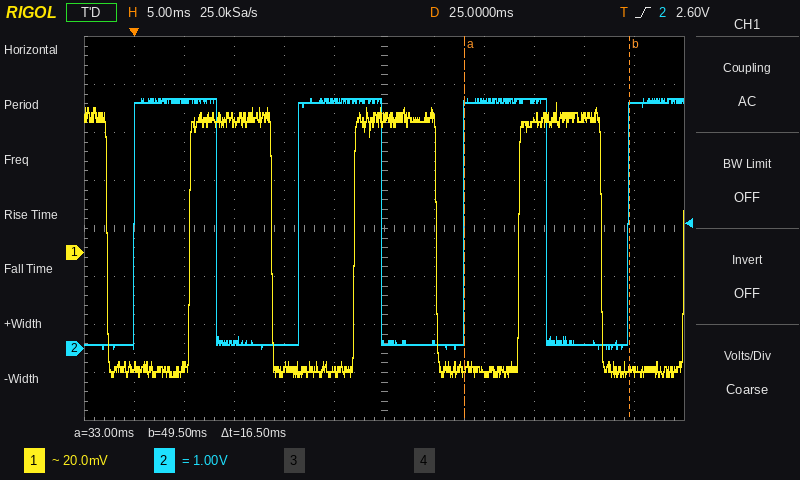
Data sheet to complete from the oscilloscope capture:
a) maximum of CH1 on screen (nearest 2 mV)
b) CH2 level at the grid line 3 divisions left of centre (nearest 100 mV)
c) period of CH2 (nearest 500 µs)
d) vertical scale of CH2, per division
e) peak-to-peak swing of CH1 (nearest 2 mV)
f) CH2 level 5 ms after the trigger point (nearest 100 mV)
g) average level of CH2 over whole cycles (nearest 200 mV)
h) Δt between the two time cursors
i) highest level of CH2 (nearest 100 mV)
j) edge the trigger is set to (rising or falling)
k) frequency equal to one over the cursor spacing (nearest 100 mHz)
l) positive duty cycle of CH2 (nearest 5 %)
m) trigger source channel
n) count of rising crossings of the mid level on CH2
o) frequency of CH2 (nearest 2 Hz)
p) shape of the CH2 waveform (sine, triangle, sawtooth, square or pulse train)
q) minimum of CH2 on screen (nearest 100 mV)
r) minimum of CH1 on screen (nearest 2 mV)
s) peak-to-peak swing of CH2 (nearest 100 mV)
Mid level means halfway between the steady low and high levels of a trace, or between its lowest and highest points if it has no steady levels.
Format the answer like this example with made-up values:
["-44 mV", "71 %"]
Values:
["62 mV", "100 mV", "16.5 ms", "1 V", "114 mV", "5.2 V", "2.6 V", "16.5 ms", "5.2 V", "rising", "60.6 Hz", "50 %", "CH2", "4", "60 Hz", "square", "0.0 V", "-52 mV", "5.2 V"]
